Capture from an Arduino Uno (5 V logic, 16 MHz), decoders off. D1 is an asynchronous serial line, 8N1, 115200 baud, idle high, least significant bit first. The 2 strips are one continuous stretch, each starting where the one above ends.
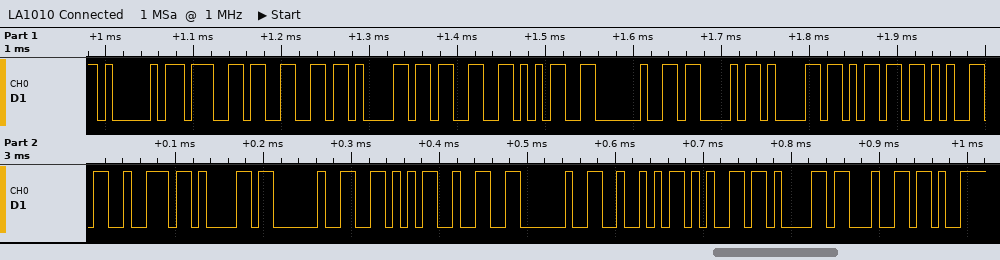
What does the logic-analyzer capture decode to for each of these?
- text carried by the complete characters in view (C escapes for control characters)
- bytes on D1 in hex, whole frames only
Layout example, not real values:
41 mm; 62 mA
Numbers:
"Agfa35 Camera V2 Read"; 41 67 66 61 33 35 20 43 61 6D 65 72 61 20 56 32 20 52 65 61 64
